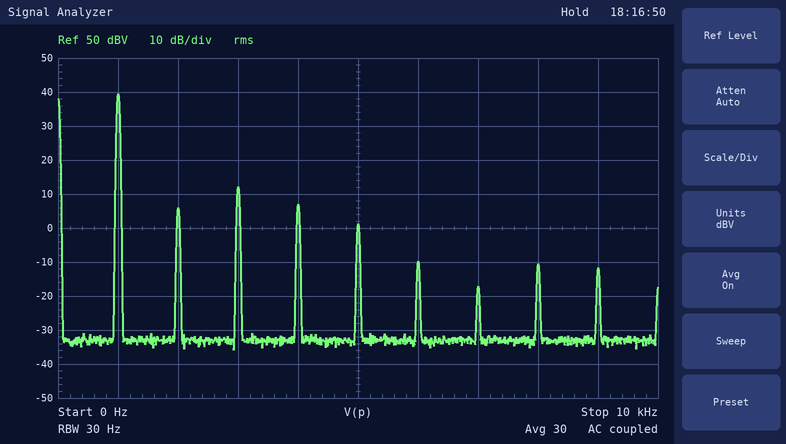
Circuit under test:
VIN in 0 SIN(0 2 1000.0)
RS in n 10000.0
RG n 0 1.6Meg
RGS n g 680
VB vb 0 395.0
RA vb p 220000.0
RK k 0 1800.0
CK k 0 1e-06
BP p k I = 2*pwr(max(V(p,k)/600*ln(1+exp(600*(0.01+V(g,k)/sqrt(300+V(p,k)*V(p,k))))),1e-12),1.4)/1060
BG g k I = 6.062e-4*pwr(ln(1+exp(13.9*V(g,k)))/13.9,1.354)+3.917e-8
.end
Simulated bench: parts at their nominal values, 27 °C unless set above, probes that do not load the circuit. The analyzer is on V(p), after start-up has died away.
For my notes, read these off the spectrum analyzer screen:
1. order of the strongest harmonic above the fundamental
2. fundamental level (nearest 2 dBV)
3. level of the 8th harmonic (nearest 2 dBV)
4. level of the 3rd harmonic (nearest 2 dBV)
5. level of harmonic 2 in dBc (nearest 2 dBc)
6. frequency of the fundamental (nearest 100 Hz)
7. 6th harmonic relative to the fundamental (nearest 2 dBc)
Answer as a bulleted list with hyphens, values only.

- 3
- 40 dBV
- -10 dBV
- 12 dBV
- -34 dBc
- 1.0 kHz
- -50 dBc
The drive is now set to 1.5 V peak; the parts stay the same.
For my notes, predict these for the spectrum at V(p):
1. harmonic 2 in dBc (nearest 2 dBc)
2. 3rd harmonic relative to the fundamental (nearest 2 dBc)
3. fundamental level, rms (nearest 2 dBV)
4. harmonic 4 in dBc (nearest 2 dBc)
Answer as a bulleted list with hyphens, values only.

- -26 dBc
- -44 dBc
- 38 dBV
- -52 dBc
